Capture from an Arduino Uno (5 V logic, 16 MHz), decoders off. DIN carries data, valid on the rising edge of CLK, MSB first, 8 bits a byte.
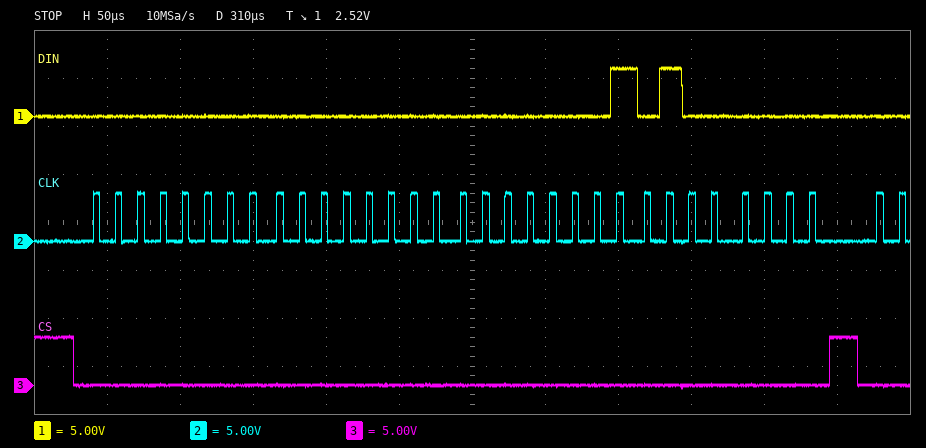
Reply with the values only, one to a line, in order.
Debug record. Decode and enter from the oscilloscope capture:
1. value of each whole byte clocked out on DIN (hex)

00 00 01 40
